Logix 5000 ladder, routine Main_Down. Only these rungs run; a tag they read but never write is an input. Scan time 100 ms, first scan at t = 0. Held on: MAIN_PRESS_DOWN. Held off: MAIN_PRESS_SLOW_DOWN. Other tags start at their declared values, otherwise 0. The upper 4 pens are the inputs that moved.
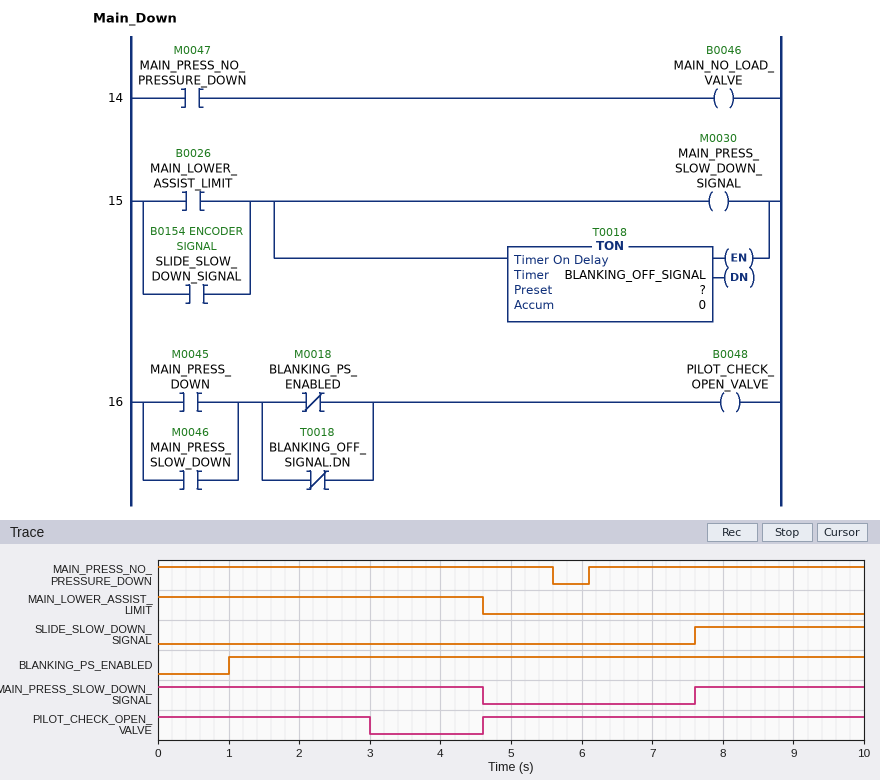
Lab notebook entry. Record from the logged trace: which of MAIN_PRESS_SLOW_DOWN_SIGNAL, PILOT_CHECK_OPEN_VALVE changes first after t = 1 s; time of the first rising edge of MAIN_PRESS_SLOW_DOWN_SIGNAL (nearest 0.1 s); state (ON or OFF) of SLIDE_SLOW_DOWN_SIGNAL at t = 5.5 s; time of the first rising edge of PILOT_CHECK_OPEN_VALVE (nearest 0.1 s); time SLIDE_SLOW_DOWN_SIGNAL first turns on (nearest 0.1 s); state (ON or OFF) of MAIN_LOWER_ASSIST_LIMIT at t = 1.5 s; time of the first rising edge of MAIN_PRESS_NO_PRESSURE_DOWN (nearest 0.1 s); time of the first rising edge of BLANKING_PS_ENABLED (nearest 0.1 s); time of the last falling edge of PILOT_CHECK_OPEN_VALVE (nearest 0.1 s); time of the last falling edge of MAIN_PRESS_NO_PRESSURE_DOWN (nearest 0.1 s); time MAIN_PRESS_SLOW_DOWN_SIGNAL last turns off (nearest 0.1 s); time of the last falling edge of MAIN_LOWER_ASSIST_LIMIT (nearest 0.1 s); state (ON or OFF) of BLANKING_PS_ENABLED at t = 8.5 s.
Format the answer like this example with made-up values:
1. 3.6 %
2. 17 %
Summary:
1. PILOT_CHECK_OPEN_VALVE
2. 7.6 s
3. OFF
4. 4.6 s
5. 7.6 s
6. ON
7. 6.1 s
8. 1.0 s
9. 3.0 s
10. 5.6 s
11. 4.6 s
12. 4.6 s
13. ON
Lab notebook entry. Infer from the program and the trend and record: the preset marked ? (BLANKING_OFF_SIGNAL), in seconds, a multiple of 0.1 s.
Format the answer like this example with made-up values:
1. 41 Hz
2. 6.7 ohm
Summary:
1. 3.0 s
